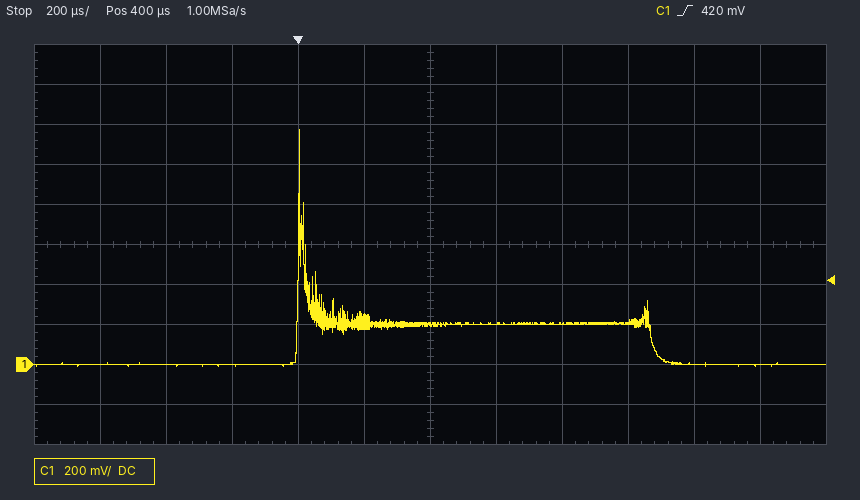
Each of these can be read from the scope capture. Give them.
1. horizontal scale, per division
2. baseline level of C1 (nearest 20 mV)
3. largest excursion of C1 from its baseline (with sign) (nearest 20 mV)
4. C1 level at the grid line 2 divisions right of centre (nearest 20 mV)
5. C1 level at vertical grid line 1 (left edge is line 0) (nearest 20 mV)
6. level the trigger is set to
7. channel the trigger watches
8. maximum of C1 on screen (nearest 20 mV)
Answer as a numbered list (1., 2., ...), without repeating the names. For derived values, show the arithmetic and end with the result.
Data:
1. 200 µs
2. 0 mV
3. 1.18 V − (0 mV) = +1.18 V
4. 200 mV
5. 0 mV
6. 420 mV
7. C1
8. 1.18 V
